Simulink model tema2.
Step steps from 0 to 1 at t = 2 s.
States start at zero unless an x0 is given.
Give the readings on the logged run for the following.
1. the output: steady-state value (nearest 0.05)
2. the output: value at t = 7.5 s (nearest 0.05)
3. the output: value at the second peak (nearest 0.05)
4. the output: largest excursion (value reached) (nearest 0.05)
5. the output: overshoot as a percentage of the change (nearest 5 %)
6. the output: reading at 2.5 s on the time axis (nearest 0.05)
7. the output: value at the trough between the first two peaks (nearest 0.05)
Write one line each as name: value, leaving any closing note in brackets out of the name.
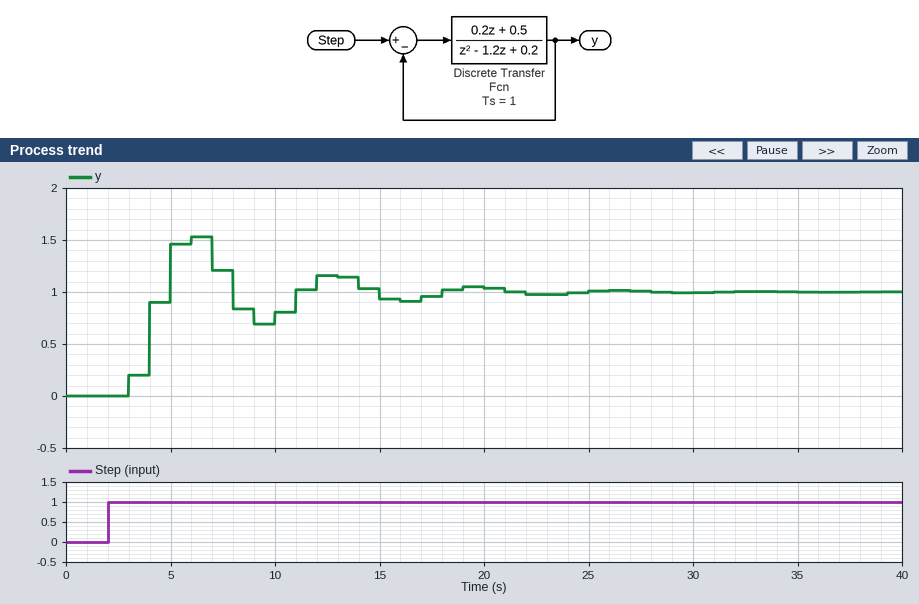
the output: steady-state value: 1.00
the output: value at t = 7.5 s: 1.20
the output: value at the second peak: 1.15
the output: largest excursion (value reached): 1.55
the output: overshoot as a percentage of the change: 55 %
the output: reading at 2.5 s on the time axis: 0.00
the output: value at the trough between the first two peaks: 0.70
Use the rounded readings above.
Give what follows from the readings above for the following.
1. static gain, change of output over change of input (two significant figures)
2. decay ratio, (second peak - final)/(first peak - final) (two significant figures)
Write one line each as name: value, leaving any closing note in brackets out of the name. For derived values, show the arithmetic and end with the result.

static gain, change of output over change of input: (1 - 0) / (1 - 0) = 1.0
decay ratio, (second peak - final)/(first peak - final): (1.15 - 1) / (1.55 - 1) = 0.27
